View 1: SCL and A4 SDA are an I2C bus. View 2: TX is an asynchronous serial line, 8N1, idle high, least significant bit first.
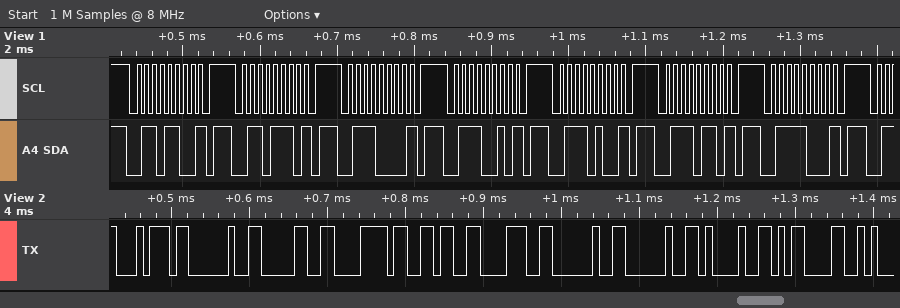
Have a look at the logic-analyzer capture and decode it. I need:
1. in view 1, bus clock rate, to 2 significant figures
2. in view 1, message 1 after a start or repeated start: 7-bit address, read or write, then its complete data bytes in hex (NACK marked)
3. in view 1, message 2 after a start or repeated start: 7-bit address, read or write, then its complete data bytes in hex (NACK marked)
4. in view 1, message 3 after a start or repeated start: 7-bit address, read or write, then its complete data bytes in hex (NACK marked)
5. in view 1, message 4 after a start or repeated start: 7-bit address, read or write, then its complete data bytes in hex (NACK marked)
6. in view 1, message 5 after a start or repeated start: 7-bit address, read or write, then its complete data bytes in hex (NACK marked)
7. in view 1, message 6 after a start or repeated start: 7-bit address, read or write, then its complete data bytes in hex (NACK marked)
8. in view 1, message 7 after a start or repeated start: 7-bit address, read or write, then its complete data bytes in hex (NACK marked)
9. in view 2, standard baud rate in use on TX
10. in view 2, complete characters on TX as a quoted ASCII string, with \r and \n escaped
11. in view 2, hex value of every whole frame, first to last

100 kHz
0x36 write NACK
0x37 write NACK
0x38 write NACK
0x39 write NACK
0x3A write NACK
0x3B write NACK
0x3C write NACK
115200 baud
"t 0x68  !\r"
74 20 30 78 36 38 20 20 21 0D
